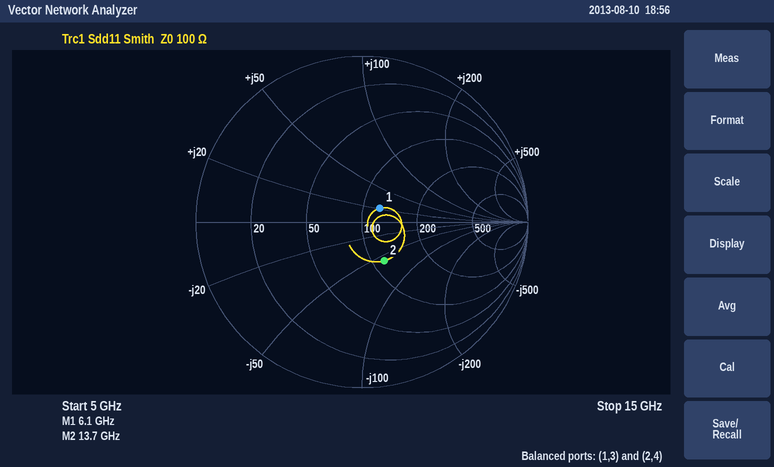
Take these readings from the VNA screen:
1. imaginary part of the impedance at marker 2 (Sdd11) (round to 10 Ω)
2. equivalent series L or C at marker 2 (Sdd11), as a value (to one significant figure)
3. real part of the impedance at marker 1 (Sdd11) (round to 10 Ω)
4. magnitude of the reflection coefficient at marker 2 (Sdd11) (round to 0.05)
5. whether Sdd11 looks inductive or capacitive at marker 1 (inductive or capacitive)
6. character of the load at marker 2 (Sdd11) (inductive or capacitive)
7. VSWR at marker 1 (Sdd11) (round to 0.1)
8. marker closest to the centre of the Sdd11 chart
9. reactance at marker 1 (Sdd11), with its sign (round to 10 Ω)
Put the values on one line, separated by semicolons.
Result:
-60 Ω; 200 fF; 120 Ω; 0.25; inductive; capacitive; 1.3; marker 1; +20 Ω
